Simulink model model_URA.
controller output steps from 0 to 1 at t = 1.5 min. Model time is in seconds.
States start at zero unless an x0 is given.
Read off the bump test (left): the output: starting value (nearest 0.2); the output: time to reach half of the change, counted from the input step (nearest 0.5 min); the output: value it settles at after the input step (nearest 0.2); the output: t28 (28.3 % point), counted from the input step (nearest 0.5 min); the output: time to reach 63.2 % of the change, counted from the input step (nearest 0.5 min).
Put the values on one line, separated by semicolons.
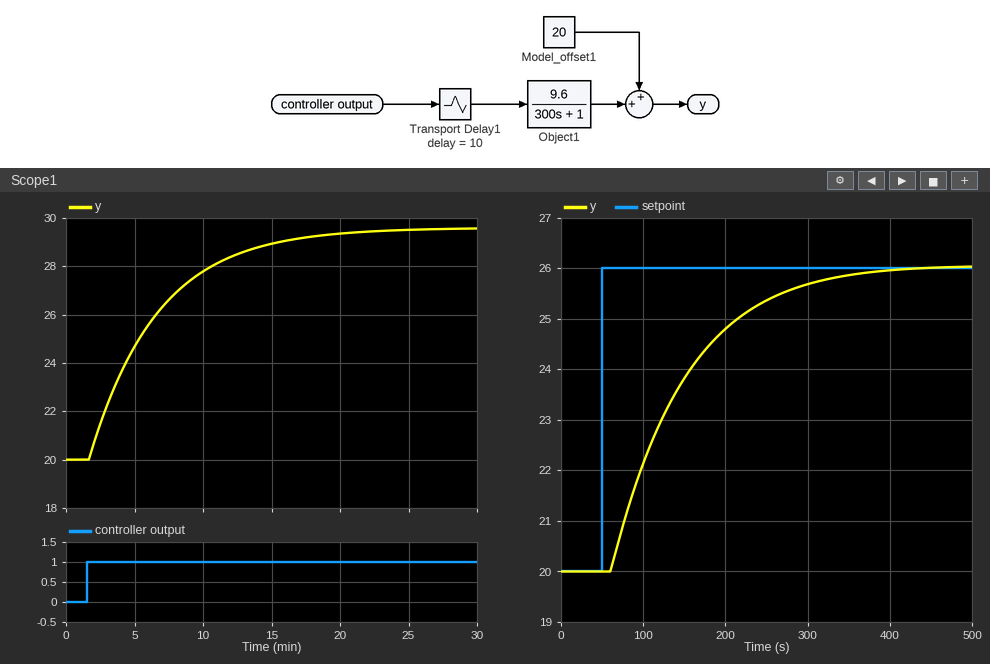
20.0; 3.5 min; 29.6; 2.0 min; 5.0 min
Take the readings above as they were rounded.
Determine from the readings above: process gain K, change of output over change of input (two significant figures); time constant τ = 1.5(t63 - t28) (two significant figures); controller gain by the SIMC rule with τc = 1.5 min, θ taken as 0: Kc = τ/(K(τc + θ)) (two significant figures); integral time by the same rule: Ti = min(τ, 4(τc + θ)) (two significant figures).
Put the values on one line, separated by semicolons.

9.6; 4.5 min; 0.31; 4.5 min
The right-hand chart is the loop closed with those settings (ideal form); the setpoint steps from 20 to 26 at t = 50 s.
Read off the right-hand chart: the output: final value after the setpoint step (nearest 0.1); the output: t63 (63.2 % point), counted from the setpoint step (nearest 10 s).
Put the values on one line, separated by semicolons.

26.0; 100 s
